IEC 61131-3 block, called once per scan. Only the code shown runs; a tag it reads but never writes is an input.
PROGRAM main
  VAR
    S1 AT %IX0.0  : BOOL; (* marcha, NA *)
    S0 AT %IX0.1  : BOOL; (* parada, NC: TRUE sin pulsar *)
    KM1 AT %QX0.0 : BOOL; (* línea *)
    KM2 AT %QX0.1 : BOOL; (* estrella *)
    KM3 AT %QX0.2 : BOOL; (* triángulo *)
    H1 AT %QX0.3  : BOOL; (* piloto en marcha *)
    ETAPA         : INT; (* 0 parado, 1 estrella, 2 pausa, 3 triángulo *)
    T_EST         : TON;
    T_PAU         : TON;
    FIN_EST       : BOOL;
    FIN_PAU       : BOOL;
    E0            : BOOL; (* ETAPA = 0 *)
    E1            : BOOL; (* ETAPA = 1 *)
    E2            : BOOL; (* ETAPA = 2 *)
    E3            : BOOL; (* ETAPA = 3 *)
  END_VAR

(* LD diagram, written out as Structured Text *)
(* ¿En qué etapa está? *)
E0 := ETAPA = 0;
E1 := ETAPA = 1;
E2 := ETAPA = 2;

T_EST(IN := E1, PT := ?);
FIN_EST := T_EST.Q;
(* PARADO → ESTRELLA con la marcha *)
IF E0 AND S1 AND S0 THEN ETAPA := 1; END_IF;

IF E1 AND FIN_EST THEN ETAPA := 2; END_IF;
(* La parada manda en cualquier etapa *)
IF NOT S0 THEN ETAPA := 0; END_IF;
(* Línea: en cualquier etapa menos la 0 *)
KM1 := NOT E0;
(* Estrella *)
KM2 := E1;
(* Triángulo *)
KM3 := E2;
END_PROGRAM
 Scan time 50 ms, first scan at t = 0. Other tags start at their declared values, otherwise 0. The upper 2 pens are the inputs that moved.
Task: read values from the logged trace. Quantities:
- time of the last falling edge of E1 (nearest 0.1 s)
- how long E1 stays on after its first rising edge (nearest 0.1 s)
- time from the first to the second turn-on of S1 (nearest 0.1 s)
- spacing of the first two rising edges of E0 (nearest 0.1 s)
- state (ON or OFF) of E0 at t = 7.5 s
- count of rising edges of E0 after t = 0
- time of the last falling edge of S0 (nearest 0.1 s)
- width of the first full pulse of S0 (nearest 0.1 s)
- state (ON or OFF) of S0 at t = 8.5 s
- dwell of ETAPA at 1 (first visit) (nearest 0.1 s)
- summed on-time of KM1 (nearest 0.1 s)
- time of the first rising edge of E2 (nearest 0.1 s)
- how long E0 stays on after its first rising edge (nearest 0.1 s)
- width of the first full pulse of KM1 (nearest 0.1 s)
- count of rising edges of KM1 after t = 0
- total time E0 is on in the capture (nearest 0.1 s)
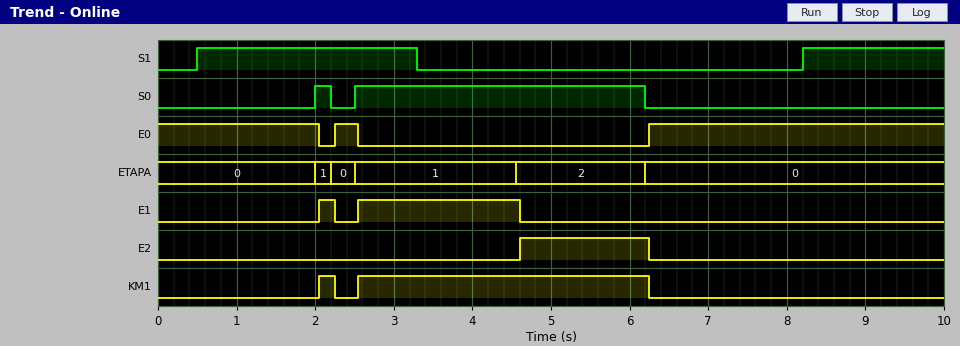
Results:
4.6 s
0.2 s
7.7 s
4.0 s
ON
2
6.2 s
0.2 s
OFF
0.2 s
3.9 s
4.6 s
0.3 s
0.2 s
2
6.1 s
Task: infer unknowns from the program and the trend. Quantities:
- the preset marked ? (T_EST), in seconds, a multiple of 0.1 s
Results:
2.0 s
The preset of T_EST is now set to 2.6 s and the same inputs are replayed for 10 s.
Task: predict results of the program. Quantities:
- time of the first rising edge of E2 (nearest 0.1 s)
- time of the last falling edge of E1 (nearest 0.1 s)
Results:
5.2 s
5.2 s
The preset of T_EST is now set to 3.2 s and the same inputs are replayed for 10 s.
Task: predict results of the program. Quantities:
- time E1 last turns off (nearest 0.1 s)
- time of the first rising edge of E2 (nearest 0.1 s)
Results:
5.8 s
5.8 s
